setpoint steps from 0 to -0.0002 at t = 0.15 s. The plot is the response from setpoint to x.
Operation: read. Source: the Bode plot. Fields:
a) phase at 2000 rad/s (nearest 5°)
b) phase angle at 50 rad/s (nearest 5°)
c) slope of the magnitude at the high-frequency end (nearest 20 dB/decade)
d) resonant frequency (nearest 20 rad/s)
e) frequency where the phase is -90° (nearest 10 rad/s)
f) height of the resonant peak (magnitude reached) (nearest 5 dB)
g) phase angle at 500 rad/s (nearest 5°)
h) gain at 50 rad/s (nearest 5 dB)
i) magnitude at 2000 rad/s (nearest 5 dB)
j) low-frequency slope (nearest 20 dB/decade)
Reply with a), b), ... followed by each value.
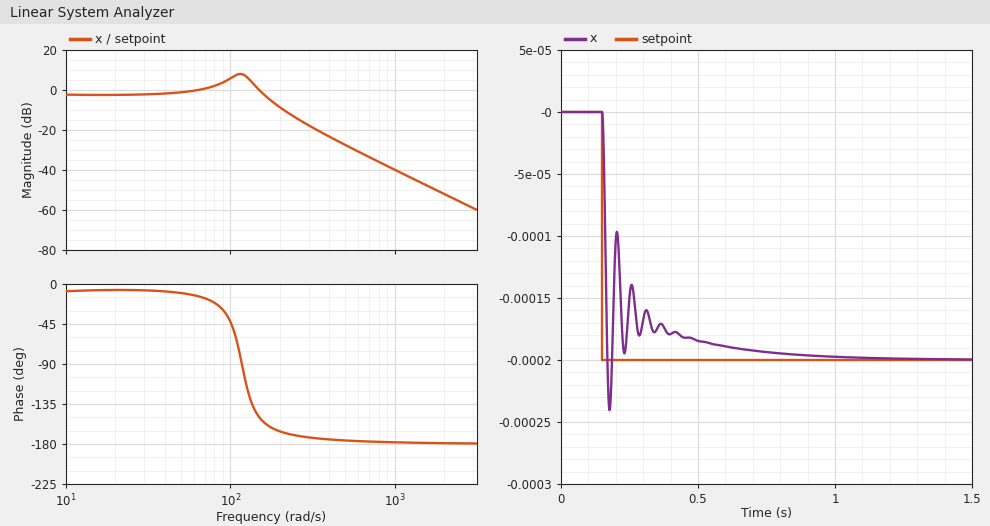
a) -180°
b) -10°
c) -40 dB/decade
d) 120 rad/s
e) 120 rad/s
f) 10 dB
g) -175°
h) 0 dB
i) -50 dB
j) 0 dB/decade
